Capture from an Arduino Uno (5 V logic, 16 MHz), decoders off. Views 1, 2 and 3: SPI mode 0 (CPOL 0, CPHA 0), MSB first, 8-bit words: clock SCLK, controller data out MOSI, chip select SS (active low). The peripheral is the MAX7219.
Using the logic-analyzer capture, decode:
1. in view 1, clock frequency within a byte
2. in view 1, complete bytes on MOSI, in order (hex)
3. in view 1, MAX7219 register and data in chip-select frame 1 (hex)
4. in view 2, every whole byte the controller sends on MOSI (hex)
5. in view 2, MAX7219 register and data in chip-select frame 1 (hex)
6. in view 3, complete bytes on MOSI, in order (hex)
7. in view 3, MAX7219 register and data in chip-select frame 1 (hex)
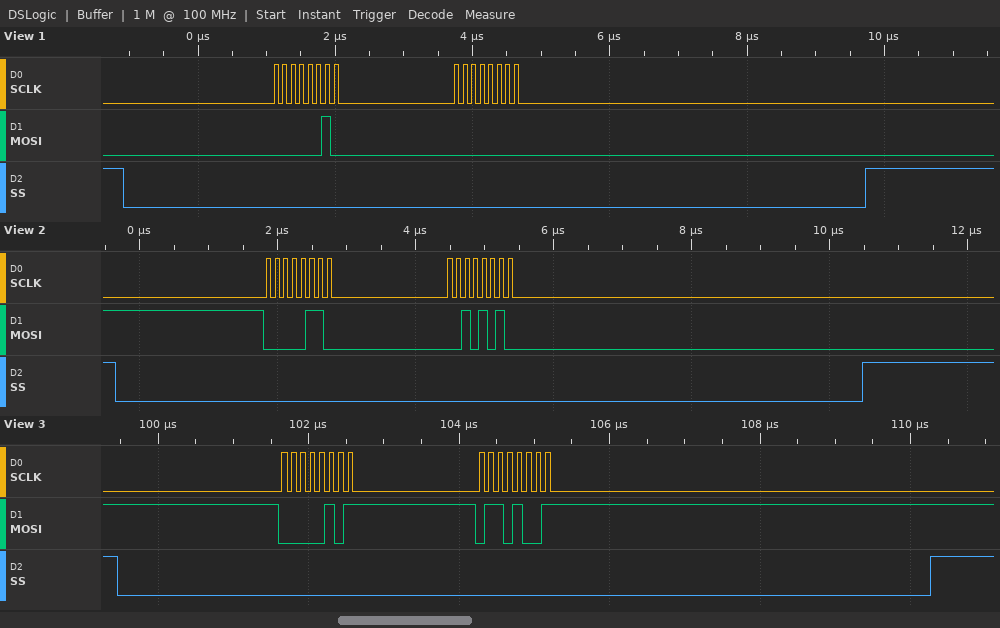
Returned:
8 MHz
0x02 0x00
register 0x2, data 0x00
0x06 0x2A
register 0x6, data 0x2A
05 69
register 0x5, data 0x69
